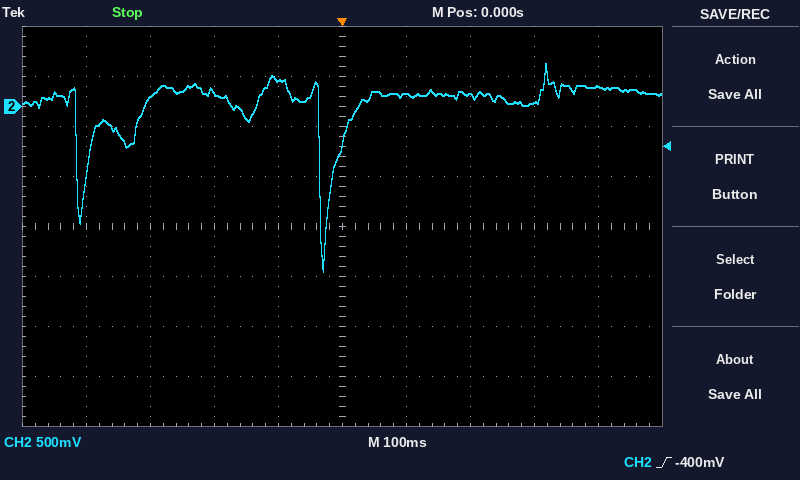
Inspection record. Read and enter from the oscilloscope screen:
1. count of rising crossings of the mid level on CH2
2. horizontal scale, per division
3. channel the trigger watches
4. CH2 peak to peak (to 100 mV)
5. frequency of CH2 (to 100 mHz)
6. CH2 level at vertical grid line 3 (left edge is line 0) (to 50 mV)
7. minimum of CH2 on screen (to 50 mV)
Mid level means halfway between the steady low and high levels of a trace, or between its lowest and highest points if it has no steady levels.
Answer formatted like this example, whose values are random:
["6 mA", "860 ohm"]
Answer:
["2", "100 ms", "CH2", "2.10 V", "2.6 Hz", "150 mV", "-1.65 V"]
